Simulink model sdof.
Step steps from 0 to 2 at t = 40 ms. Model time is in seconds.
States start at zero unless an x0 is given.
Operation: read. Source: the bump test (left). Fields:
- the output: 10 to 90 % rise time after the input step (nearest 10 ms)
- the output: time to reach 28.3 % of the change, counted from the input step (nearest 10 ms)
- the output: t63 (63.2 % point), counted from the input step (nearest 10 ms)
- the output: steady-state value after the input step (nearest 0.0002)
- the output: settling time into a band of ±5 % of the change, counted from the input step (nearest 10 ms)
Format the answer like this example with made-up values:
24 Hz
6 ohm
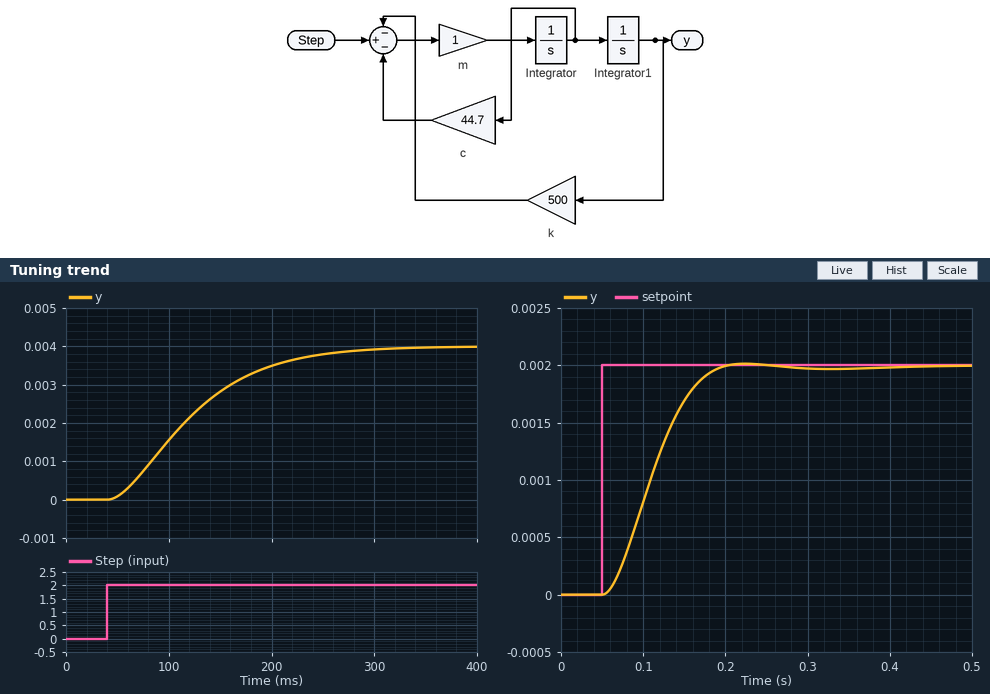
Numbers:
150 ms
50 ms
100 ms
0.0040
210 ms
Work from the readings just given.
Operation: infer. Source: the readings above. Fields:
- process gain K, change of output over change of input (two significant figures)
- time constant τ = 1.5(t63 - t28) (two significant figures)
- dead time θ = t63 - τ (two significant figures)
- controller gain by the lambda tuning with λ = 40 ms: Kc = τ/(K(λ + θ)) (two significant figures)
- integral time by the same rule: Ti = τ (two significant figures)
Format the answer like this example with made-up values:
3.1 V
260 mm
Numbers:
0.0020
75 ms
25 ms
580
75 ms
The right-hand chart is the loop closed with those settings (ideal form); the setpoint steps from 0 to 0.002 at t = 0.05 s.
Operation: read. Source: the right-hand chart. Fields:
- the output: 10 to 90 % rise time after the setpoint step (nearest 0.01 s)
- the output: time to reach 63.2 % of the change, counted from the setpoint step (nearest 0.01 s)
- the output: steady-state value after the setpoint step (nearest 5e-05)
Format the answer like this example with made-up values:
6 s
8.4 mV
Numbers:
0.09 s
0.07 s
0.00200
